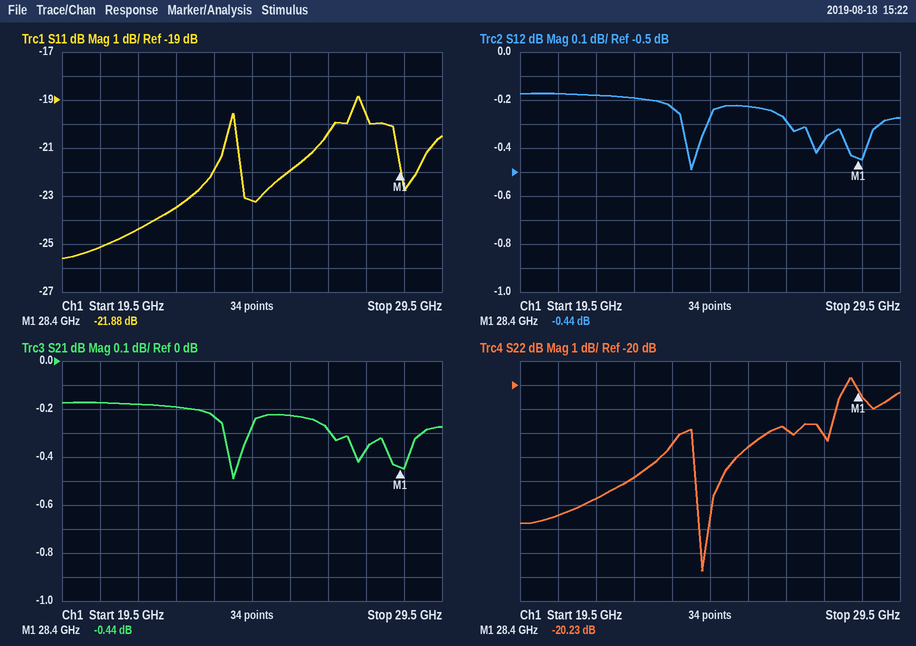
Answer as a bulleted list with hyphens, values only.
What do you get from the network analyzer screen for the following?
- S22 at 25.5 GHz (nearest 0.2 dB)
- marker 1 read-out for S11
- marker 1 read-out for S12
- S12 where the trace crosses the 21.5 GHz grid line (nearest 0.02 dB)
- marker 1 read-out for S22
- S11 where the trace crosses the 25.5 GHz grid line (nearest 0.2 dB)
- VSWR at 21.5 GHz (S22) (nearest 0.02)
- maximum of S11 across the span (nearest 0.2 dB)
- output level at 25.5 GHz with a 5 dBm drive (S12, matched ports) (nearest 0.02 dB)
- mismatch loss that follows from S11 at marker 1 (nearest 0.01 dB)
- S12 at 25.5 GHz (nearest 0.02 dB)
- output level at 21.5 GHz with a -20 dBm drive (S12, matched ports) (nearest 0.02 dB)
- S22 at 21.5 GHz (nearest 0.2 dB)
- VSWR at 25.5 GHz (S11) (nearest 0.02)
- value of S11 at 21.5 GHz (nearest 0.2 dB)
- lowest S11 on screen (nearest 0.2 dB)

- -22.6 dB
- -21.88 dB
- -0.44 dB
- -0.18 dB
- -20.23 dB
- -22.0 dB
- 1.12
- -18.8 dB
- 4.78 dBm
- 0.03 dB
- -0.22 dB
- -20.18 dBm
- -24.8 dB
- 1.18
- -24.4 dB
- -25.6 dB
